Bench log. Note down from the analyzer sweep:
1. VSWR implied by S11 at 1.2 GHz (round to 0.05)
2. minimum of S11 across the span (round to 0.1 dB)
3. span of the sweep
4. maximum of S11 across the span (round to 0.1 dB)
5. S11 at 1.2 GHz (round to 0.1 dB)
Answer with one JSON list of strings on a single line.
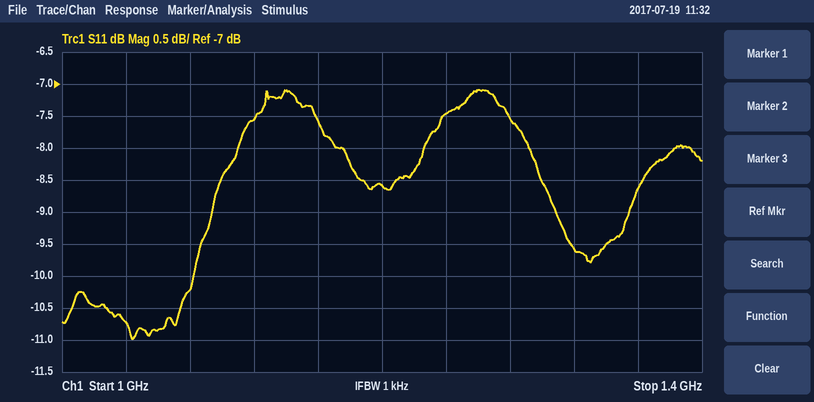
["2.20", "-11.0 dB", "400 MHz", "-7.1 dB", "-8.6 dB"]
